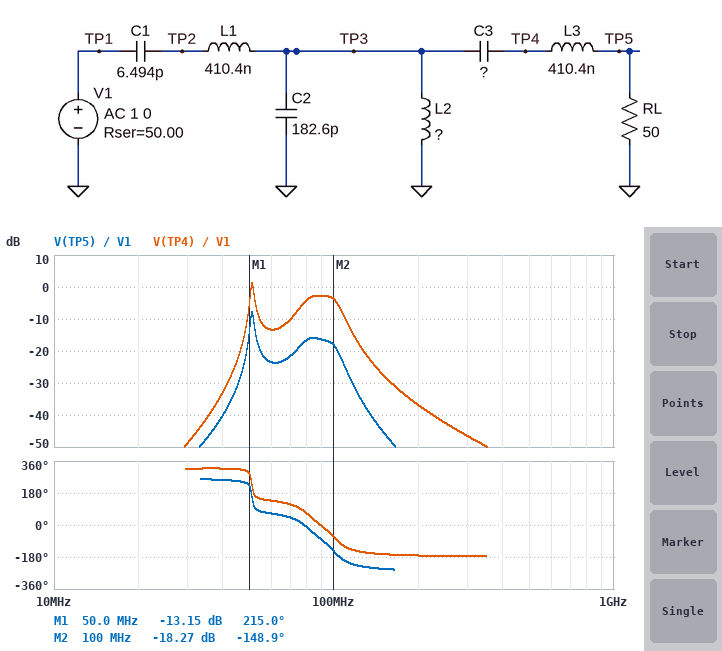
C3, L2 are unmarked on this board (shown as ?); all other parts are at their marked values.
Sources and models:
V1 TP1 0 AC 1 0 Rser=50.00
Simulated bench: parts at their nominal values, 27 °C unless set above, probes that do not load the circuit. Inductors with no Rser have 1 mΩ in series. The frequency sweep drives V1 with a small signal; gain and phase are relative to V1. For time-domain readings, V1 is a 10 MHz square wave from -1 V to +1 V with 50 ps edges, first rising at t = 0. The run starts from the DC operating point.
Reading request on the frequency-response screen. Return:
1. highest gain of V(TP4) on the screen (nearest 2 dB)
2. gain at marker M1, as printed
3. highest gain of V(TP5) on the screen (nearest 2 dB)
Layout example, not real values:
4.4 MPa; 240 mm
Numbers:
2 dB; -13.15 dB; -8 dB
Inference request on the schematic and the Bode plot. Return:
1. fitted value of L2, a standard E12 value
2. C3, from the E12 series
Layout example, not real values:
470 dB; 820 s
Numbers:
47 nH; 10 pF
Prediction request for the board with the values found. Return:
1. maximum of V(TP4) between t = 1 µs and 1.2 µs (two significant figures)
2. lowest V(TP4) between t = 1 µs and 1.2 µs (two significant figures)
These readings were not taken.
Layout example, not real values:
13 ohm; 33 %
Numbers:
340 mV; -340 mV
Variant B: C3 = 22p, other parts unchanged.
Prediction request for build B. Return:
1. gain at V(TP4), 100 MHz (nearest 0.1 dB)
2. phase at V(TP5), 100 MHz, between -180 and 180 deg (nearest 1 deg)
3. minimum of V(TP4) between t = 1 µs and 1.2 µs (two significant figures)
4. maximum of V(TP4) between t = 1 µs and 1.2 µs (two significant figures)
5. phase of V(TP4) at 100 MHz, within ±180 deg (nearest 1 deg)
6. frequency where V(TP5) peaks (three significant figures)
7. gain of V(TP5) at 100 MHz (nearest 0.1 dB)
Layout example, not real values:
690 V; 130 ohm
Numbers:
-8.9 dB; -163 deg; -210 mV; 210 mV; -84 deg; 60.3 MHz; -23.3 dB
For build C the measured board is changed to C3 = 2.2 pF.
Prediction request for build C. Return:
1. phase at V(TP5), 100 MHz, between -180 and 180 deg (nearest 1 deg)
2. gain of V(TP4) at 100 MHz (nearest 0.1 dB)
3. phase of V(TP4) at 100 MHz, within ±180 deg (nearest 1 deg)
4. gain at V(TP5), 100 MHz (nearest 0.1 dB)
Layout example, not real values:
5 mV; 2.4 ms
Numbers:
-7 deg; -17.4 dB; 72 deg; -31.8 dB
